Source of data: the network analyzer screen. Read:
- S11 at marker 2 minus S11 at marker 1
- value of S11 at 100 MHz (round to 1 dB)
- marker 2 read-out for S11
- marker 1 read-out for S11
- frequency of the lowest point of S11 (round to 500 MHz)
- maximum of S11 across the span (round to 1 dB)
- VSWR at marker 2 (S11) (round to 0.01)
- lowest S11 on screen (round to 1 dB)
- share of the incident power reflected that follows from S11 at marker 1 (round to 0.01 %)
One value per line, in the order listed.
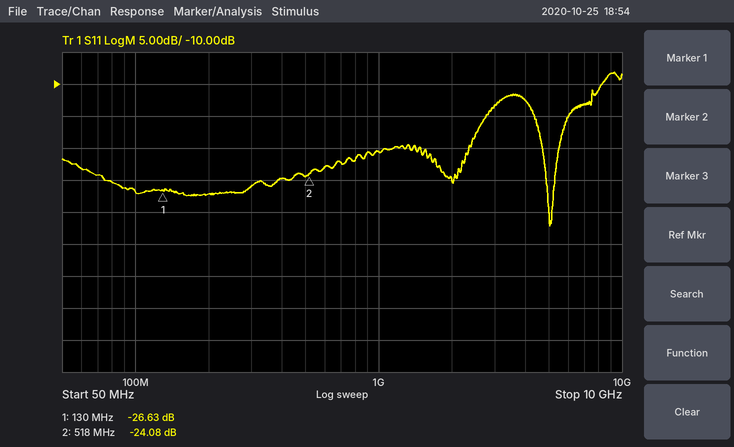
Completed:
2.55 dB
-27 dB
-24.08 dB
-26.63 dB
5.0 GHz
-8 dB
1.13
-32 dB
0.22 %
